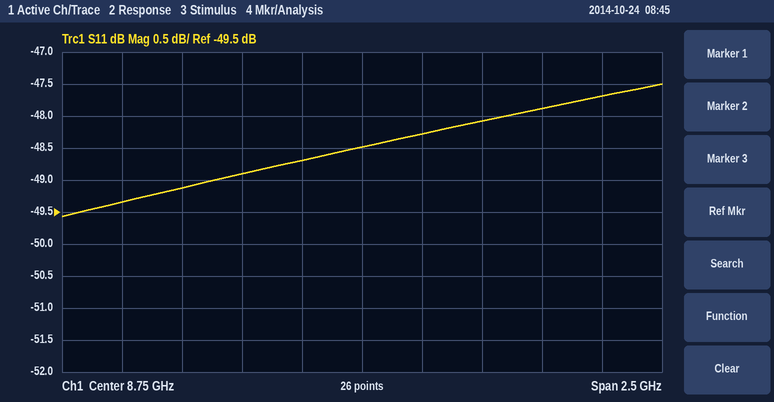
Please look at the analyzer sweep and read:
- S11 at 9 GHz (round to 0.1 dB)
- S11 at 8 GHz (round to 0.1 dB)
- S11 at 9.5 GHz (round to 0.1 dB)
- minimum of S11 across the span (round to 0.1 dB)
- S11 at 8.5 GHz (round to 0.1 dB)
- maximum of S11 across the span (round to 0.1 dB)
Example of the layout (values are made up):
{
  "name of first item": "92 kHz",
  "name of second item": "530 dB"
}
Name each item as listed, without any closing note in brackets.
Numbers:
{
  "S11 at 9 GHz": "-48.3 dB",
  "S11 at 8 GHz": "-49.1 dB",
  "S11 at 9.5 GHz": "-47.9 dB",
  "minimum of S11 across the span": "-49.6 dB",
  "S11 at 8.5 GHz": "-48.7 dB",
  "maximum of S11 across the span": "-47.5 dB"
}
